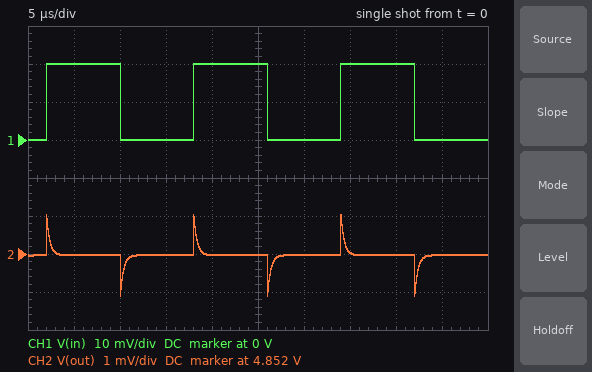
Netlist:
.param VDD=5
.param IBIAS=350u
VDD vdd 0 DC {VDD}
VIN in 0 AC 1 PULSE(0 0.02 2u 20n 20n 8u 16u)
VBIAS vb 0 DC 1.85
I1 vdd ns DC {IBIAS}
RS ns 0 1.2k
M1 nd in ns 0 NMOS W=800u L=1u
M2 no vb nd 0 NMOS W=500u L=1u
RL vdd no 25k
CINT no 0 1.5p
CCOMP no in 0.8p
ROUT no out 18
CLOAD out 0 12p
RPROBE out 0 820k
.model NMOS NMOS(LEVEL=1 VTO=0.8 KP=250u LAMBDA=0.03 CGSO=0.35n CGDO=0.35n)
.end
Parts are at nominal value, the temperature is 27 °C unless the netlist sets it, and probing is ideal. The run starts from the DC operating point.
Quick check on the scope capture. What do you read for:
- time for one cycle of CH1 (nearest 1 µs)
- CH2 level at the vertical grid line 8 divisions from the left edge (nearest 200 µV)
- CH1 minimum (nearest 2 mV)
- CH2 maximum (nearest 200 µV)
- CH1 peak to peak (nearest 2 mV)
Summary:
16 µs
4.8520 V
0 V
4.8530 V
20 mV
